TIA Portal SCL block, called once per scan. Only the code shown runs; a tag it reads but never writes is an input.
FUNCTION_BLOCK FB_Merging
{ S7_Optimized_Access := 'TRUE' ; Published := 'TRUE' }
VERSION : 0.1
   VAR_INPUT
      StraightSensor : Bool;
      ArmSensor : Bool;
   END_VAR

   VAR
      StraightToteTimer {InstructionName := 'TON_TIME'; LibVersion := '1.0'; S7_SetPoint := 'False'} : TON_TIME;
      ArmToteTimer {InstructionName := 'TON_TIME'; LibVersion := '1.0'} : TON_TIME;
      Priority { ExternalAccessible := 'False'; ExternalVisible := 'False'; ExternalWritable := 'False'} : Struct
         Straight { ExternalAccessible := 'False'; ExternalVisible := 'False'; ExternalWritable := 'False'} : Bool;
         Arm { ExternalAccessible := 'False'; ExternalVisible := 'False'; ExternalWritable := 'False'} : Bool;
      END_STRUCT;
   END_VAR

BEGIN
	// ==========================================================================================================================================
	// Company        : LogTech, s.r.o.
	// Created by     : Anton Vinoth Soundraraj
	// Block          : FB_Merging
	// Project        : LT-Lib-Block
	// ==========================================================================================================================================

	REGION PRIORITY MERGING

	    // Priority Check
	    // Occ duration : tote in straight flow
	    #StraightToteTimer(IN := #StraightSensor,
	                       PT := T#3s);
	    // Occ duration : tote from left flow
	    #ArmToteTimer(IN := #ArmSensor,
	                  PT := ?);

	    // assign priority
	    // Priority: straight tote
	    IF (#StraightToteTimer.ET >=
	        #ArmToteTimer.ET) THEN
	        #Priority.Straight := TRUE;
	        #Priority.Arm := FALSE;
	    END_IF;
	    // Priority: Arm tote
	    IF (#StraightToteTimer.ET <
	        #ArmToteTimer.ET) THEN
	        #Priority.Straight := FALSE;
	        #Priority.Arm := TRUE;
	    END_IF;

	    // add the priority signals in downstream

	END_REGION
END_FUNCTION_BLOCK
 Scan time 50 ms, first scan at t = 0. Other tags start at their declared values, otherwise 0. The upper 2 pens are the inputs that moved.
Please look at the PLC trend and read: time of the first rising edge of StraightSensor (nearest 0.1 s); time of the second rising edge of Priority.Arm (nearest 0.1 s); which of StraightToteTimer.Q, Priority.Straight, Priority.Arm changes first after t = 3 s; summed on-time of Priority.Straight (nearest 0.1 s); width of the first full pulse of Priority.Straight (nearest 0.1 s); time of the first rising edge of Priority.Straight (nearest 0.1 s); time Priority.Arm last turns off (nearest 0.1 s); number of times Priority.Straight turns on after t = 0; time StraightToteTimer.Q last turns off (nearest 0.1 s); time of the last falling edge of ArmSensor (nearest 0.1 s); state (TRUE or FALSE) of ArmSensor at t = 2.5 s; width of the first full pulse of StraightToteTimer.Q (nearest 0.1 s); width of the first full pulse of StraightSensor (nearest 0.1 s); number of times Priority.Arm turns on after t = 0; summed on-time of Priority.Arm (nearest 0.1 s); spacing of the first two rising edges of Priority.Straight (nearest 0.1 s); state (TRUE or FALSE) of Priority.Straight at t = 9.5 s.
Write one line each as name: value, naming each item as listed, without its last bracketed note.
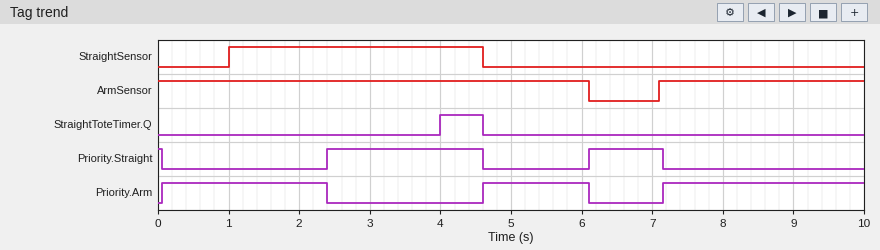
time of the first rising edge of StraightSensor: 1.0 s
time of the second rising edge of Priority.Arm: 4.6 s
which of StraightToteTimer.Q, Priority.Straight, Priority.Arm changes first after t = 3 s: StraightToteTimer.Q
summed on-time of Priority.Straight: 3.3 s
width of the first full pulse of Priority.Straight: 2.2 s
time of the first rising edge of Priority.Straight: 2.4 s
time Priority.Arm last turns off: 6.1 s
number of times Priority.Straight turns on after t = 0: 2
time StraightToteTimer.Q last turns off: 4.6 s
time of the last falling edge of ArmSensor: 6.1 s
state (TRUE or FALSE) of ArmSensor at t = 2.5 s: TRUE
width of the first full pulse of StraightToteTimer.Q: 0.6 s
width of the first full pulse of StraightSensor: 3.6 s
number of times Priority.Arm turns on after t = 0: 3
summed on-time of Priority.Arm: 6.7 s
spacing of the first two rising edges of Priority.Straight: 3.7 s
state (TRUE or FALSE) of Priority.Straight at t = 9.5 s: FALSE
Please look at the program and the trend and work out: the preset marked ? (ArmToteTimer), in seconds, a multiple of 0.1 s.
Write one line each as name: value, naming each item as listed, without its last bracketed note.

the preset marked ? (ArmToteTimer), in seconds, a multiple of 0.1 s: 1.4 s
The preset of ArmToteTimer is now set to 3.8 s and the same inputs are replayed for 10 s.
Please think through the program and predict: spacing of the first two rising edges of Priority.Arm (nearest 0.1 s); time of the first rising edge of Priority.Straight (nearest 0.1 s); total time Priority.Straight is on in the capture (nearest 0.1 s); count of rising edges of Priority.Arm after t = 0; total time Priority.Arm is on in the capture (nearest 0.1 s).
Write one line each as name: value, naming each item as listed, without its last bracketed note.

spacing of the first two rising edges of Priority.Arm: 7.1 s
time of the first rising edge of Priority.Straight: 6.1 s
total time Priority.Straight is on in the capture: 1.1 s
count of rising edges of Priority.Arm after t = 0: 2
total time Priority.Arm is on in the capture: 8.9 s
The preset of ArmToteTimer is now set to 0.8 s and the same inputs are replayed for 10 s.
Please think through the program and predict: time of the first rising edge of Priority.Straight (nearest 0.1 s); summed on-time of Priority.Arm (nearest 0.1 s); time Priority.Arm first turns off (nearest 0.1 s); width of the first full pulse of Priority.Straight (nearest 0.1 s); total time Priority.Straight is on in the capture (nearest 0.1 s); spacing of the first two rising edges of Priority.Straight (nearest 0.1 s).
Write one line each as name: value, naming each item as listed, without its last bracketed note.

time of the first rising edge of Priority.Straight: 1.8 s
summed on-time of Priority.Arm: 6.1 s
time Priority.Arm first turns off: 1.8 s
width of the first full pulse of Priority.Straight: 2.8 s
total time Priority.Straight is on in the capture: 3.9 s
spacing of the first two rising edges of Priority.Straight: 4.3 s
